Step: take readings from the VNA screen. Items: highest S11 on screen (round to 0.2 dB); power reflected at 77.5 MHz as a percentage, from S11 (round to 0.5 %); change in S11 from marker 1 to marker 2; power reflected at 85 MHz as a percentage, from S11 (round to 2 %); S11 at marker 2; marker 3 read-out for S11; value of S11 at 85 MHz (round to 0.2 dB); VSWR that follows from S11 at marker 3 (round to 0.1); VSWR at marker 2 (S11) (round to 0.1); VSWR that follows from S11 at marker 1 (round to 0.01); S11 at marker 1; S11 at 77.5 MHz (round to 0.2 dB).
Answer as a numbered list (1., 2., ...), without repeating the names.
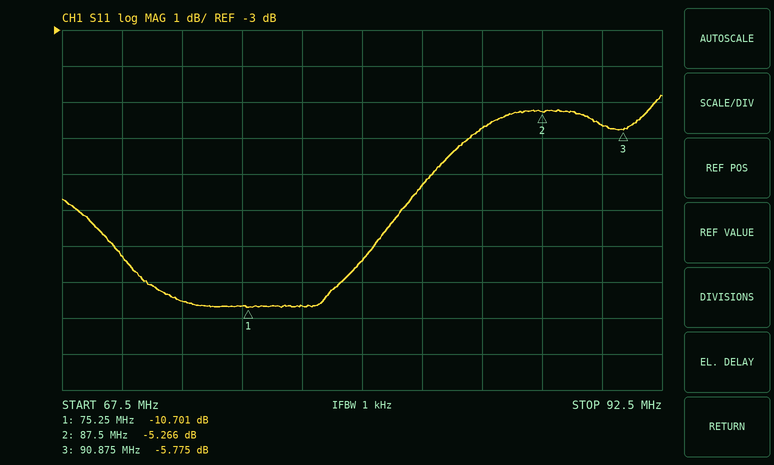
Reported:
1. -4.8 dB
2. 8.5 %
3. 5.435 dB
4. 26 %
5. -5.266 dB
6. -5.775 dB
7. -5.8 dB
8. 3.1
9. 3.4
10. 1.82
11. -10.701 dB
12. -10.6 dB
